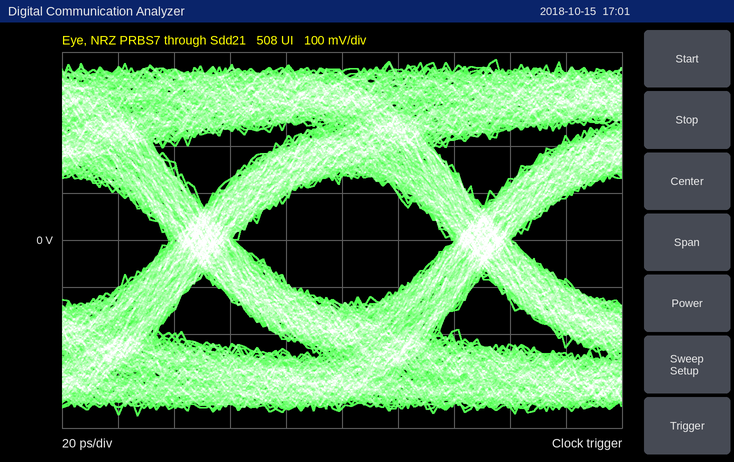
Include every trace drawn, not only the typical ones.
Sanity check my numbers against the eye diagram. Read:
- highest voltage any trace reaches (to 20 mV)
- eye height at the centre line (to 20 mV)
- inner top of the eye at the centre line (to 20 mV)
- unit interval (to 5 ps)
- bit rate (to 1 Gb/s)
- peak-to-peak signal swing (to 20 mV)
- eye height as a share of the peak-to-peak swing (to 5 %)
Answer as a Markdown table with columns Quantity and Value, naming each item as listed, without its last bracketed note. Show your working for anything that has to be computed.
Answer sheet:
| Quantity | Value |
|---|---|
| highest voltage any trace reaches | 380 mV |
| eye height at the centre line | 280 mV |
| inner top of the eye at the centre line | 140 mV |
| unit interval | 100 ps |
| bit rate | 10 Gb/s |
| peak-to-peak signal swing | 760 mV |
| eye height as a share of the peak-to-peak swing | 280 mV / 760 mV ≈ 36.8 %, so 35 % to the nearest 5 % |
